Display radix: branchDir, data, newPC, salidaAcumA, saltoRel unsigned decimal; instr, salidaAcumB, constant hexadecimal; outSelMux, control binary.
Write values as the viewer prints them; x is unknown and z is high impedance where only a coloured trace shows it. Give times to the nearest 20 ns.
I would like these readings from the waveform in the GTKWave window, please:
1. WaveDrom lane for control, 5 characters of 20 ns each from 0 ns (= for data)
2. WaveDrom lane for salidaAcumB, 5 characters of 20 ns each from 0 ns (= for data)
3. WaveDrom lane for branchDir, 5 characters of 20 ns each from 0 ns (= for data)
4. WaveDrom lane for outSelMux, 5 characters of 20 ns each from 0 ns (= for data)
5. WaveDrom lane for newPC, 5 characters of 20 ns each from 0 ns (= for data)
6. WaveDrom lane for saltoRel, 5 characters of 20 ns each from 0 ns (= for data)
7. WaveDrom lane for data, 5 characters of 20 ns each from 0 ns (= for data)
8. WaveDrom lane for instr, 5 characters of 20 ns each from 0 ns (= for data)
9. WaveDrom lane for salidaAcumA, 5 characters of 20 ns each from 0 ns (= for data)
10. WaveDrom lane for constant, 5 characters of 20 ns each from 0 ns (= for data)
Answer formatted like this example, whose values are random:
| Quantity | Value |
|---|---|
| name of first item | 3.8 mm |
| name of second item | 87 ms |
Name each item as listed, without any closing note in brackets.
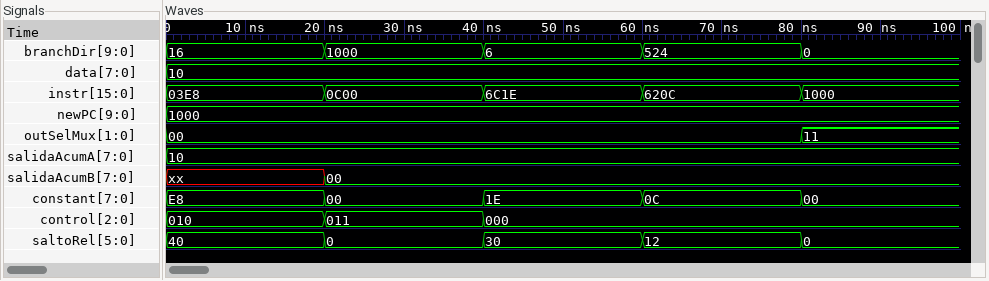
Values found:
| Quantity | Value |
|---|---|
| WaveDrom lane for control, 5 characters of 20 ns each from 0 ns | {name: 'control', wave: '===..', data: '010 011 000'} |
| WaveDrom lane for salidaAcumB, 5 characters of 20 ns each from 0 ns | {name: 'salidaAcumB', wave: 'x=...', data: '00'} |
| WaveDrom lane for branchDir, 5 characters of 20 ns each from 0 ns | {name: 'branchDir', wave: '=====', data: '16 1000 6 524 0'} |
| WaveDrom lane for outSelMux, 5 characters of 20 ns each from 0 ns | {name: 'outSelMux', wave: '=...=', data: '00 11'} |
| WaveDrom lane for newPC, 5 characters of 20 ns each from 0 ns | {name: 'newPC', wave: '=....', data: '1000'} |
| WaveDrom lane for saltoRel, 5 characters of 20 ns each from 0 ns | {name: 'saltoRel', wave: '=====', data: '40 0 30 12 0'} |
| WaveDrom lane for data, 5 characters of 20 ns each from 0 ns | {name: 'data', wave: '=....', data: '10'} |
| WaveDrom lane for instr, 5 characters of 20 ns each from 0 ns | {name: 'instr', wave: '=====', data: '03E8 0C00 6C1E 620C 1000'} |
| WaveDrom lane for salidaAcumA, 5 characters of 20 ns each from 0 ns | {name: 'salidaAcumA', wave: '=....', data: '10'} |
| WaveDrom lane for constant, 5 characters of 20 ns each from 0 ns | {name: 'constant', wave: '=====', data: 'E8 00 1E 0C 00'} |
